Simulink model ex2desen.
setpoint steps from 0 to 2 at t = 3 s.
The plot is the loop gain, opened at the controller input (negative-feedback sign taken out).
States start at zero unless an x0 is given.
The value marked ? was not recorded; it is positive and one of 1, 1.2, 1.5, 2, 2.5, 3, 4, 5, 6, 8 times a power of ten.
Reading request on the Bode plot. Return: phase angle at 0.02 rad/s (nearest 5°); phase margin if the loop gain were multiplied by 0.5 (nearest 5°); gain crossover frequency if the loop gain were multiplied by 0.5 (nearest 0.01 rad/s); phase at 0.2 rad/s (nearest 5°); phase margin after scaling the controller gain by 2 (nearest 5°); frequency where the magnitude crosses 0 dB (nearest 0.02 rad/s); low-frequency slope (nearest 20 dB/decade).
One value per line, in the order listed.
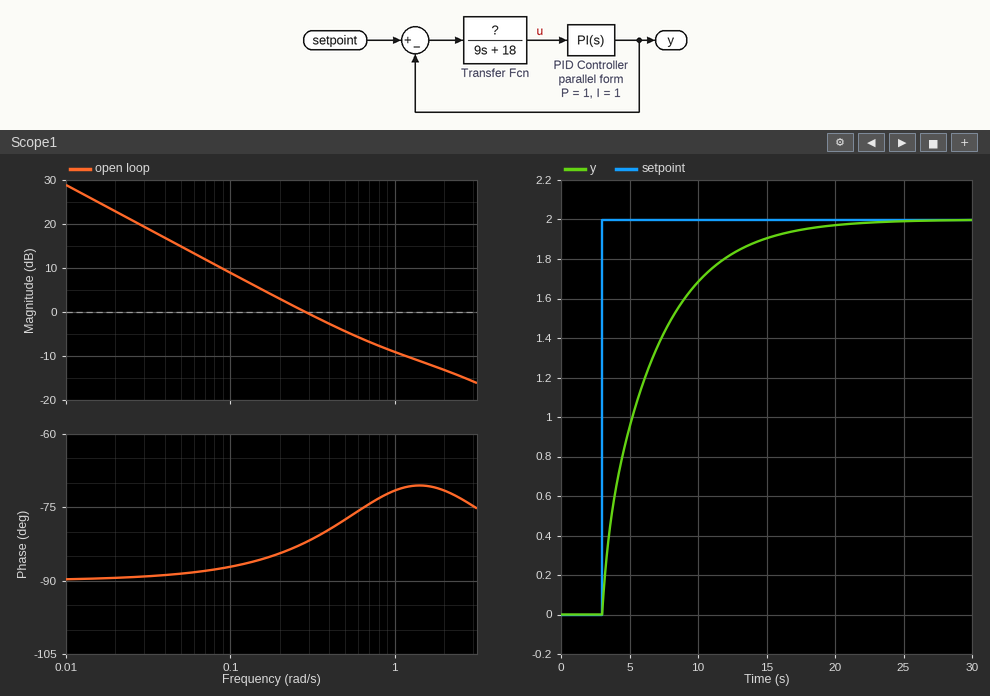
-90°
95°
0.14 rad/s
-85°
105°
0.28 rad/s
-20 dB/decade
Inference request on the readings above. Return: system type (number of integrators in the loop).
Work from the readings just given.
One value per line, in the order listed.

1
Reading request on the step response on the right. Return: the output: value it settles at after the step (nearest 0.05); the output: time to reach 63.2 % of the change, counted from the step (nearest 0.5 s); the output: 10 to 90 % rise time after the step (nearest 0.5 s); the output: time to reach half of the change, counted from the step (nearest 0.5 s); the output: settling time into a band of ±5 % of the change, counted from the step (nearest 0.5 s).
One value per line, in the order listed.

2.00
3.5 s
8.5 s
2.0 s
12.0 s
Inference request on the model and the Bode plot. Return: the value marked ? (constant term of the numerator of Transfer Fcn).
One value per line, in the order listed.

5
